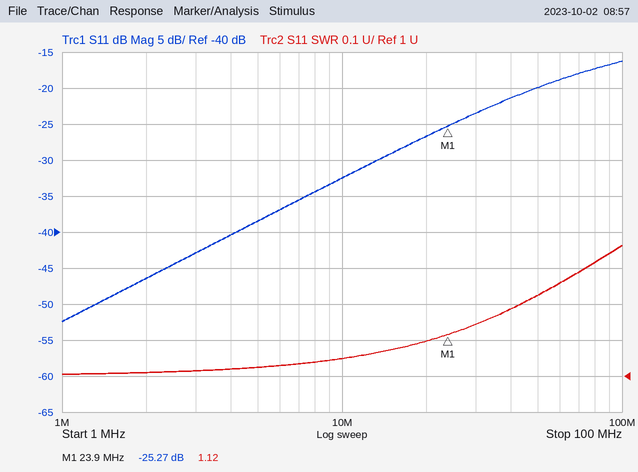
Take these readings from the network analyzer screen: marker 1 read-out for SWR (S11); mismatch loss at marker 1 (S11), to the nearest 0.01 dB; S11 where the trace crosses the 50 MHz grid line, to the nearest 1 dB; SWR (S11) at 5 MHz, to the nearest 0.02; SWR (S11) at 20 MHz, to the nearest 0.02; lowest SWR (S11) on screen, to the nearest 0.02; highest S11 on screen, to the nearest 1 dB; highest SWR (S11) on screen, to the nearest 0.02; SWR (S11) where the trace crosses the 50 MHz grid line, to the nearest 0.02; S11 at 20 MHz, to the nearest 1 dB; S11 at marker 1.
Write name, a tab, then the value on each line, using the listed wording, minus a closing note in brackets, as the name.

marker 1 read-out for SWR	1.12
mismatch loss at marker 1 (S11), to the nearest 0.01 dB	0.01 dB
S11 where the trace crosses the 50 MHz grid line, to the nearest 1 dB	-20 dB
SWR (S11) at 5 MHz, to the nearest 0.02	1.02
SWR (S11) at 20 MHz, to the nearest 0.02	1.10
lowest SWR (S11) on screen, to the nearest 0.02	1.00
highest S11 on screen, to the nearest 1 dB	-16 dB
highest SWR (S11) on screen, to the nearest 0.02	1.36
SWR (S11) where the trace crosses the 50 MHz grid line, to the nearest 0.02	1.22
S11 at 20 MHz, to the nearest 1 dB	-27 dB
S11 at marker 1	-25.27 dB
